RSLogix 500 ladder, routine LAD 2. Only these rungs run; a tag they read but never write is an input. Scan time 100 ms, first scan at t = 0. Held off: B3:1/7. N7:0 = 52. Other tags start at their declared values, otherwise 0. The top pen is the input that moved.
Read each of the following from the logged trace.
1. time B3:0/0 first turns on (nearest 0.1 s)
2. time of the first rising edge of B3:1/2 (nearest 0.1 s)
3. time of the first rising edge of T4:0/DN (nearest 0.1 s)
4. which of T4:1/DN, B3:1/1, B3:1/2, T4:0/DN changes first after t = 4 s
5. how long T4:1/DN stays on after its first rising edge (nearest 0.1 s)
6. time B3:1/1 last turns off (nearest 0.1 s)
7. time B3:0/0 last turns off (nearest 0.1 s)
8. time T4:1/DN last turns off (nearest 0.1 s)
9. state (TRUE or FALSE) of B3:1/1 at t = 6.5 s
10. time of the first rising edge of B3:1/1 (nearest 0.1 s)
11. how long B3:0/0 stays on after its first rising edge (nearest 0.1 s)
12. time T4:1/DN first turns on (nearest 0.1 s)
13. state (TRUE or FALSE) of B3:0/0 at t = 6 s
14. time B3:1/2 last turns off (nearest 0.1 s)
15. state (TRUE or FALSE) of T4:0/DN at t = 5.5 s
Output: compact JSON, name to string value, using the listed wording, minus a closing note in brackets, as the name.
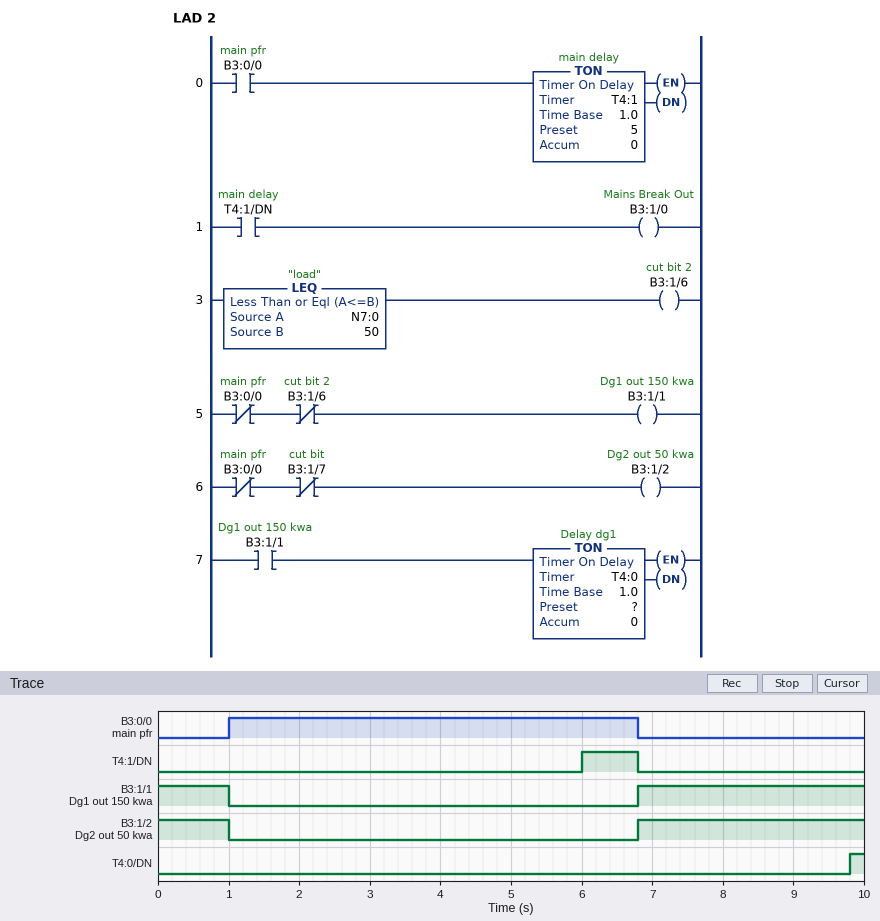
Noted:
{"time B3:0/0 first turns on": "1.0 s", "time of the first rising edge of B3:1/2": "6.8 s", "time of the first rising edge of T4:0/DN": "9.8 s", "which of T4:1/DN, B3:1/1, B3:1/2, T4:0/DN changes first after t = 4 s": "T4:1/DN", "how long T4:1/DN stays on after its first rising edge": "0.8 s", "time B3:1/1 last turns off": "1.0 s", "time B3:0/0 last turns off": "6.8 s", "time T4:1/DN last turns off": "6.8 s", "state (TRUE or FALSE) of B3:1/1 at t = 6.5 s": "FALSE", "time of the first rising edge of B3:1/1": "6.8 s", "how long B3:0/0 stays on after its first rising edge": "5.8 s", "time T4:1/DN first turns on": "6.0 s", "state (TRUE or FALSE) of B3:0/0 at t = 6 s": "TRUE", "time B3:1/2 last turns off": "1.0 s", "state (TRUE or FALSE) of T4:0/DN at t = 5.5 s": "FALSE"}
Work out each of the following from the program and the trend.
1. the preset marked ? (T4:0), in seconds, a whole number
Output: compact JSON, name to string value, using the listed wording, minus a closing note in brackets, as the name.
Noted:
{"the preset marked ? (T4:0), in seconds, a whole number": "3 s"}
